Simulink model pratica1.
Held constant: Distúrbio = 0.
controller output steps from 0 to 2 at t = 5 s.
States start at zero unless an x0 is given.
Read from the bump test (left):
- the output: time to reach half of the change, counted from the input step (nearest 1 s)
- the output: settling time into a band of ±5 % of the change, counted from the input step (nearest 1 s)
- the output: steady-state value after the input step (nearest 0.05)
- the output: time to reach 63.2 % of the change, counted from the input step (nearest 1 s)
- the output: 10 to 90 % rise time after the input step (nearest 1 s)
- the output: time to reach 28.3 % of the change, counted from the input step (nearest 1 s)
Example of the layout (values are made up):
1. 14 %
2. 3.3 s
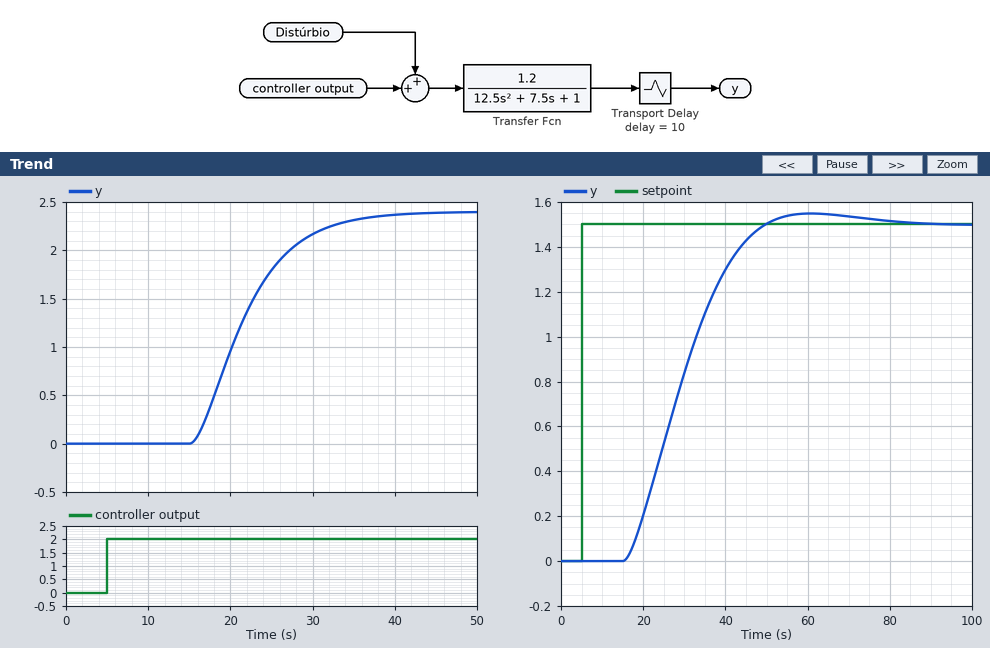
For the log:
1. 16 s
2. 28 s
3. 2.40
4. 18 s
5. 13 s
6. 14 s
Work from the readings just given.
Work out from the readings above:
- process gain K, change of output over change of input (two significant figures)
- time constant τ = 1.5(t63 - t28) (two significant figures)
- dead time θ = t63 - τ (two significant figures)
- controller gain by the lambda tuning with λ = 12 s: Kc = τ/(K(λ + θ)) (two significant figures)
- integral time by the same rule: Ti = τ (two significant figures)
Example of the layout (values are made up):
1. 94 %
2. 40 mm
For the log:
1. 1.2
2. 6.0 s
3. 12 s
4. 0.21
5. 6.0 s
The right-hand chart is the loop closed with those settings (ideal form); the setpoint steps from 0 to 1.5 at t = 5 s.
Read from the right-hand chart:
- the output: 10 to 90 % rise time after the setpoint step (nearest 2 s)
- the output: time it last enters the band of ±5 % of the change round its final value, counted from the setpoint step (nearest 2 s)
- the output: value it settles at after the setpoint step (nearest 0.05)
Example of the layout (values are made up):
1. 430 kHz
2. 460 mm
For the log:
1. 22 s
2. 40 s
3. 1.50
